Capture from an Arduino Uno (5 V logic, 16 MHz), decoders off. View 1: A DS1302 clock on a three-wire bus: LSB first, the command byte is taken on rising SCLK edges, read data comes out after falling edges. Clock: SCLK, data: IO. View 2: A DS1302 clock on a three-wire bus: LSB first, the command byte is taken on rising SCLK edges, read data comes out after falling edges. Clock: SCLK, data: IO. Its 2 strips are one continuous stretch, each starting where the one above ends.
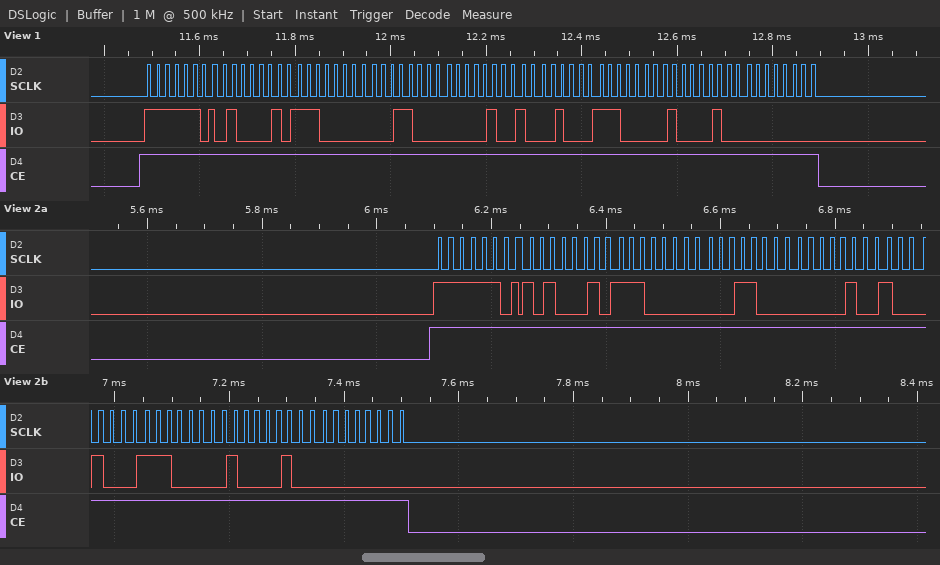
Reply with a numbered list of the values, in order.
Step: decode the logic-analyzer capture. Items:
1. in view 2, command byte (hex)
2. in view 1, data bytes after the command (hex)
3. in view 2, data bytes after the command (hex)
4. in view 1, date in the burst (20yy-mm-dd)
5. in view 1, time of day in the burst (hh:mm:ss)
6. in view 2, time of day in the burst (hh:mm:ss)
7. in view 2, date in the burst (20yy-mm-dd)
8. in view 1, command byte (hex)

1. 0xBF
2. 42 07 18 20 11 07 21 00
3. 45 07 18 20 11 07 21 00
4. 2021-11-20
5. 18:07:42
6. 18:07:45
7. 2021-11-20
8. 0xBF
